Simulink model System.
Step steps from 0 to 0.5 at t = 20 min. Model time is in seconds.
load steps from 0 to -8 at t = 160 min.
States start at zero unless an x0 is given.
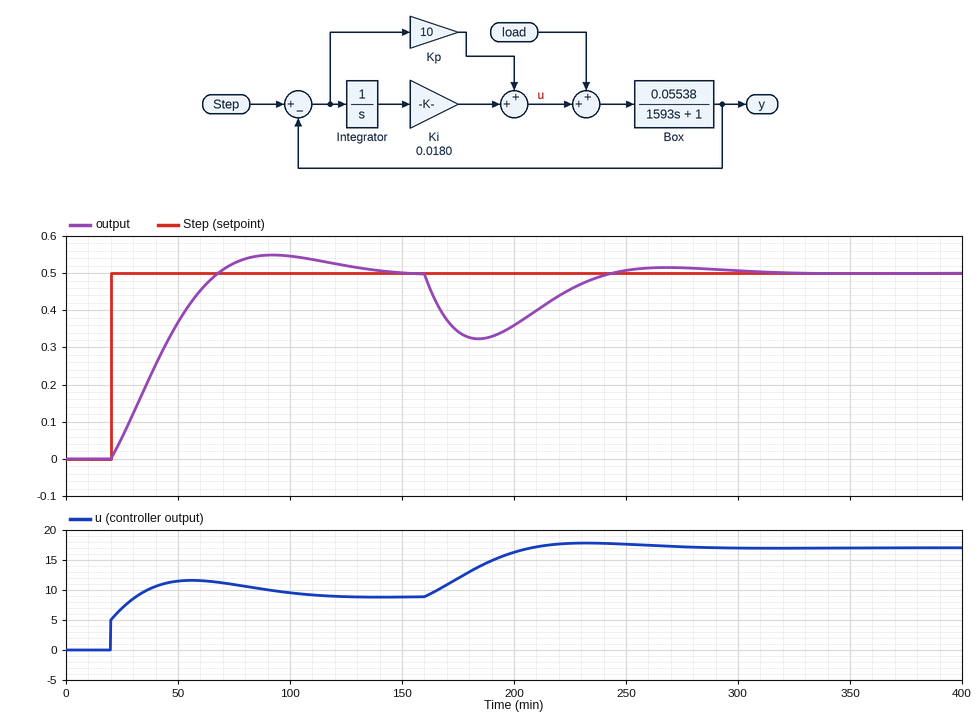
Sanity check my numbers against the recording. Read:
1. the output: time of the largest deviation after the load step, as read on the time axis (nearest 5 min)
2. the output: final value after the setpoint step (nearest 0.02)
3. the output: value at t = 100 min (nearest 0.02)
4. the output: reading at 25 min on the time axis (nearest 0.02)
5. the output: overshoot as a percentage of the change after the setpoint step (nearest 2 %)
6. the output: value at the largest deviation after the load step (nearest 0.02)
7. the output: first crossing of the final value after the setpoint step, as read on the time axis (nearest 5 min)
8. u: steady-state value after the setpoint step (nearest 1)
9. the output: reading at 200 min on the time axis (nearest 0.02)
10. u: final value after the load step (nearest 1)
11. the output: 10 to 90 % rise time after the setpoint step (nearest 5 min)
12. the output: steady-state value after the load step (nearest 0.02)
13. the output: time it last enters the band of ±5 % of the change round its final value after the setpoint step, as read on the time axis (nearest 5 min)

185 min
0.50
0.54
0.06
10 %
0.32
70 min
9
0.36
17
35 min
0.50
120 min
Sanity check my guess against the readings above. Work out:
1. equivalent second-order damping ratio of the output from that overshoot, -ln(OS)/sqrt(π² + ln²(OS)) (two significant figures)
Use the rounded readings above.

0.59
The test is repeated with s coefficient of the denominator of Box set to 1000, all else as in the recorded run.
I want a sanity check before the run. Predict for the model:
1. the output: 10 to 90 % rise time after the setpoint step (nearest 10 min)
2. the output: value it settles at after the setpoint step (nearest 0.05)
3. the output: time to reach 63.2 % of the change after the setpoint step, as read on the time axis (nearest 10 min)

30 min
0.50
40 min
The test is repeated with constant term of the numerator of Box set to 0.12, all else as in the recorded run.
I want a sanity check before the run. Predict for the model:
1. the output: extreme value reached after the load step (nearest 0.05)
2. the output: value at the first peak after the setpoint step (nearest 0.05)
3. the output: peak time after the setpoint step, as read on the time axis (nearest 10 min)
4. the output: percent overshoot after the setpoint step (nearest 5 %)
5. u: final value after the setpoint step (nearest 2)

0.25
0.55
60 min
15 %
4
